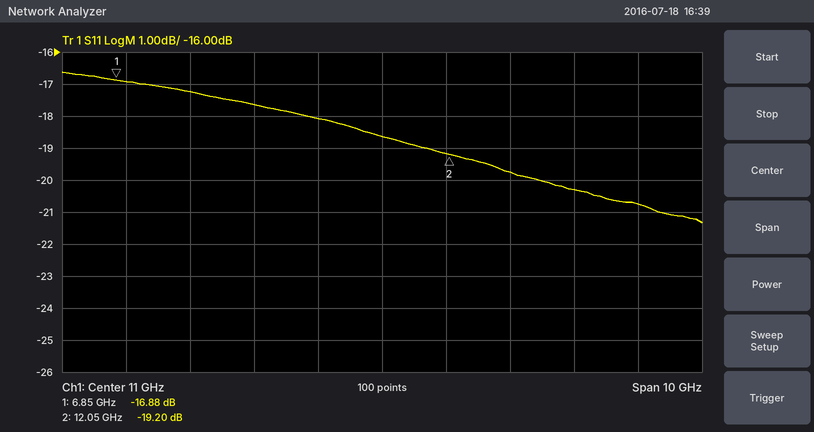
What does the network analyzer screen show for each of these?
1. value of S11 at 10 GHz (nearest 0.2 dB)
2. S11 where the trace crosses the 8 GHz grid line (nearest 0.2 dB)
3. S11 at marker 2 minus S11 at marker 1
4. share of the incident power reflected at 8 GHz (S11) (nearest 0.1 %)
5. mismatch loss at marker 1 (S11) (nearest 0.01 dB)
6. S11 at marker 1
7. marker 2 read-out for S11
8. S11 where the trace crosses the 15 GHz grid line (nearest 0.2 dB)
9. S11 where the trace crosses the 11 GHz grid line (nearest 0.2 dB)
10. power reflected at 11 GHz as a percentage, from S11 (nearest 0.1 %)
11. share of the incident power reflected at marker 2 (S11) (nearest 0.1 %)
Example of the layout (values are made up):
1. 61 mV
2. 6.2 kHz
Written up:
1. -18.0 dB
2. -17.2 dB
3. -2.32 dB
4. 1.9 %
5. 0.09 dB
6. -16.88 dB
7. -19.20 dB
8. -20.8 dB
9. -18.6 dB
10. 1.4 %
11. 1.2 %
